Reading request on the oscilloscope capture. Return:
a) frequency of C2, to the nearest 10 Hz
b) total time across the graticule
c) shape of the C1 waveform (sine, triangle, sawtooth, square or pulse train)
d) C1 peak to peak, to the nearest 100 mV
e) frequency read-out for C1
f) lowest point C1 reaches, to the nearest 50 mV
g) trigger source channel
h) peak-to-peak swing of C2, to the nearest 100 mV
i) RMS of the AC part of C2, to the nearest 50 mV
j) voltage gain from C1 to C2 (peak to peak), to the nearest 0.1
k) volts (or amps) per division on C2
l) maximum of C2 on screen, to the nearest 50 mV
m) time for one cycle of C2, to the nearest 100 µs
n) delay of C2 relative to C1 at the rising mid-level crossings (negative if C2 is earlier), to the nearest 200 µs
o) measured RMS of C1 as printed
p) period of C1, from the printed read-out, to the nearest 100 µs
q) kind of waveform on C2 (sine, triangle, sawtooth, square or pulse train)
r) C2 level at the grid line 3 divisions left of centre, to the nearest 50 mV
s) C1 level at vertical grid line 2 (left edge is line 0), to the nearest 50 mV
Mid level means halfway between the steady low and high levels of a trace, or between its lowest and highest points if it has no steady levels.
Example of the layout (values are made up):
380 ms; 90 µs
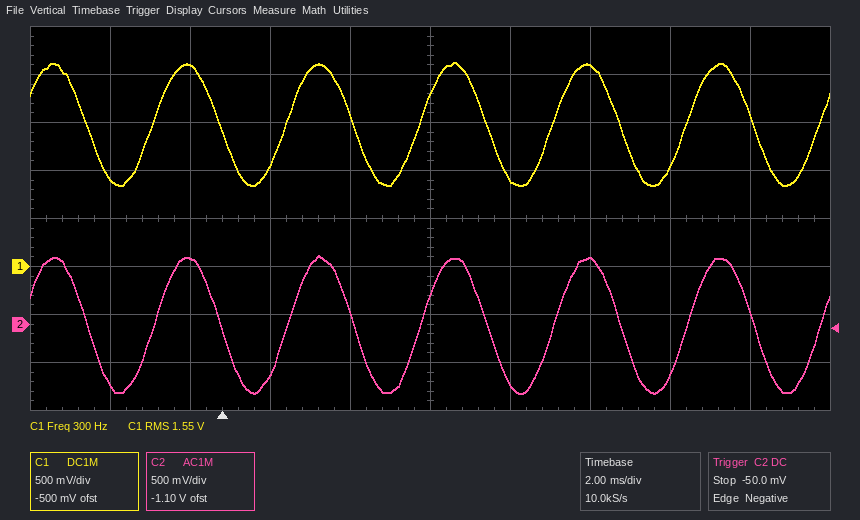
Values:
300 Hz; 20 ms; sine; 1.30 V; 300 Hz; 850 mV; C2; 1.40 V; 500 mV; 1.1; 500 mV; 700 mV; 3.3 ms; 0.0 ms; 1.55 V; 3.3 ms; sine; 700 mV; 2.10 V
